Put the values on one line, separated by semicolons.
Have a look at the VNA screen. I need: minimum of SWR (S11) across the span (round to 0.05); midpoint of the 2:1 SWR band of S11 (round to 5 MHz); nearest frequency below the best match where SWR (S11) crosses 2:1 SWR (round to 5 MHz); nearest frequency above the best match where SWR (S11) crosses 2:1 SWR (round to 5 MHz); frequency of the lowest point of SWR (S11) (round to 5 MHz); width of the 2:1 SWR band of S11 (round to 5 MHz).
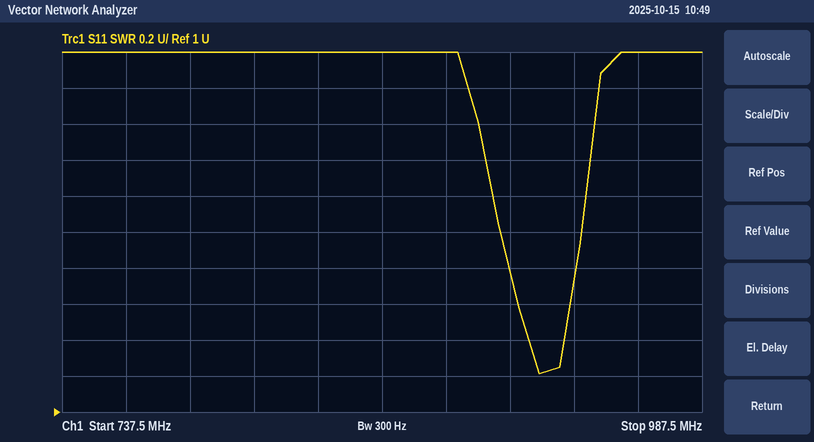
1.20; 925 MHz; 910 MHz; 940 MHz; 925 MHz; 30 MHz
